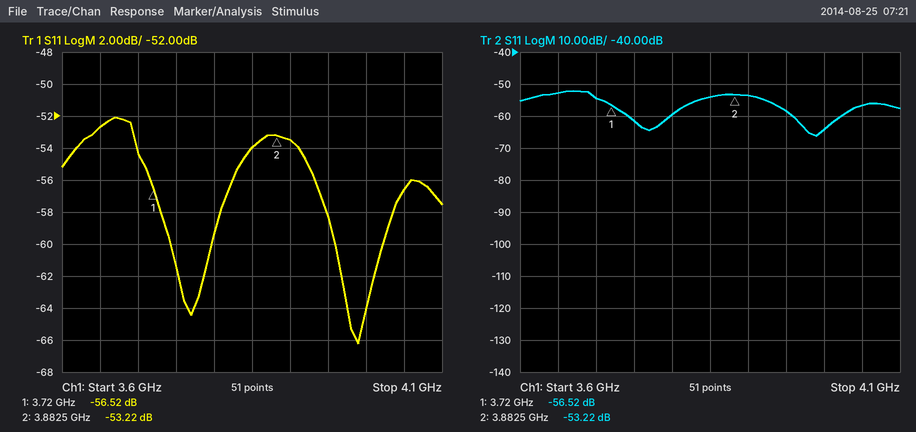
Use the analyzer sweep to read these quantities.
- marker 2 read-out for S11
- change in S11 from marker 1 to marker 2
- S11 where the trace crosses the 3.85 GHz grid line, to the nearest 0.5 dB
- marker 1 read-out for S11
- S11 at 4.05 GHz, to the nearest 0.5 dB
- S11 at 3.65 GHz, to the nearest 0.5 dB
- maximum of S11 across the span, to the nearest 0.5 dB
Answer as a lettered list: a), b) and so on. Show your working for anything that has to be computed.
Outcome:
a) -53.22 dB
b) -53.22 − (-56.52) = 3.30 dB
c) -54.0 dB
d) -56.52 dB
e) -56.5 dB
f) -52.5 dB
g) -52.0 dB
